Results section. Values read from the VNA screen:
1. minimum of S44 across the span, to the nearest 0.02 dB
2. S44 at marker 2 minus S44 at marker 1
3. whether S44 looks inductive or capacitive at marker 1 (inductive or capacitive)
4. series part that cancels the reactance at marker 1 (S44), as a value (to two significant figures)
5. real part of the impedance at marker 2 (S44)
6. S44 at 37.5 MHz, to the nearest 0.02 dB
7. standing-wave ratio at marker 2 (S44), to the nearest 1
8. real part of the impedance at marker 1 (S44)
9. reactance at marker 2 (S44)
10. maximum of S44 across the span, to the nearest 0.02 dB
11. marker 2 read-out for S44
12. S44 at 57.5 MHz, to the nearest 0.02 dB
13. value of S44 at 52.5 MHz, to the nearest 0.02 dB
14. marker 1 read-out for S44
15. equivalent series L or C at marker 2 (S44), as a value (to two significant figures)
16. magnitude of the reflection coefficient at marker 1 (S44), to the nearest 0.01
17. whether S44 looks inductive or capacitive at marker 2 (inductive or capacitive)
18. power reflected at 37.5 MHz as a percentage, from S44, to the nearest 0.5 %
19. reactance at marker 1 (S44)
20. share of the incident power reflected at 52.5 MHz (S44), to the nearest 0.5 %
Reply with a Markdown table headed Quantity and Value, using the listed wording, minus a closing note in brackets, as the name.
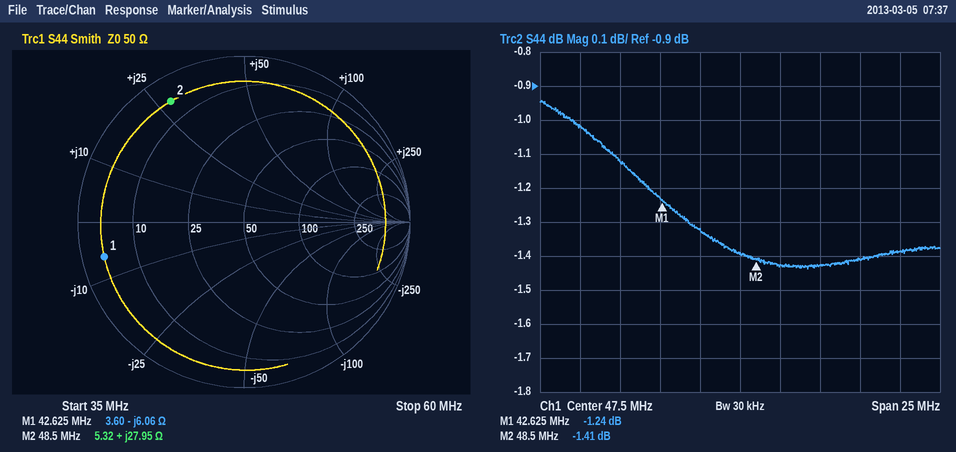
| Quantity | Value |
|---|---|
| minimum of S44 across the span, to the nearest 0.02 dB | -1.44 dB |
| S44 at marker 2 minus S44 at marker 1 | -0.17 dB |
| whether S44 looks inductive or capacitive at marker 1 | capacitive |
| series part that cancels the reactance at marker 1 (S44), as a value | 23 nH |
| real part of the impedance at marker 2 | 5.32 Ω |
| S44 at 37.5 MHz, to the nearest 0.02 dB | -1.02 dB |
| standing-wave ratio at marker 2 (S44), to the nearest 1 | 12 |
| real part of the impedance at marker 1 | 3.60 Ω |
| reactance at marker 2 | +27.95 Ω |
| maximum of S44 across the span, to the nearest 0.02 dB | -0.94 dB |
| marker 2 read-out for S44 | -1.41 dB |
| S44 at 57.5 MHz, to the nearest 0.02 dB | -1.38 dB |
| value of S44 at 52.5 MHz, to the nearest 0.02 dB | -1.42 dB |
| marker 1 read-out for S44 | -1.24 dB |
| equivalent series L or C at marker 2 (S44), as a value | 92 nH |
| magnitude of the reflection coefficient at marker 1 (S44), to the nearest 0.01 | 0.87 |
| whether S44 looks inductive or capacitive at marker 2 | inductive |
| power reflected at 37.5 MHz as a percentage, from S44, to the nearest 0.5 % | 79.0 % |
| reactance at marker 1 | -6.06 Ω |
| share of the incident power reflected at 52.5 MHz (S44), to the nearest 0.5 % | 72.0 % |
